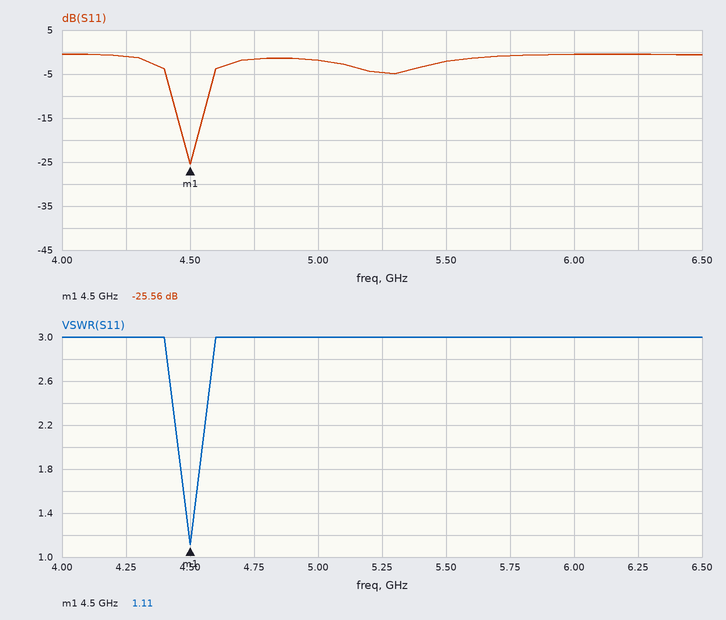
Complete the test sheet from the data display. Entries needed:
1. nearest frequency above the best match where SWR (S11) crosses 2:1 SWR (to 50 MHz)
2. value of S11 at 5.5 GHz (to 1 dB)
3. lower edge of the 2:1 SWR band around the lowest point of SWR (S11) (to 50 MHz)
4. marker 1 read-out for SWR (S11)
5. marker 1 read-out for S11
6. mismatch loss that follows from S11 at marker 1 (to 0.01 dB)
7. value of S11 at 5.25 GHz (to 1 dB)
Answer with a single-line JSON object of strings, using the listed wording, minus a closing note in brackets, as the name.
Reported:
{"nearest frequency above the best match where SWR (S11) crosses 2:1 SWR": "4.55 GHz", "value of S11 at 5.5 GHz": "-2 dB", "lower edge of the 2:1 SWR band around the lowest point of SWR (S11)": "4.45 GHz", "marker 1 read-out for SWR": "1.11", "marker 1 read-out for S11": "-25.56 dB", "mismatch loss that follows from S11 at marker 1": "0.01 dB", "value of S11 at 5.25 GHz": "-5 dB"}
